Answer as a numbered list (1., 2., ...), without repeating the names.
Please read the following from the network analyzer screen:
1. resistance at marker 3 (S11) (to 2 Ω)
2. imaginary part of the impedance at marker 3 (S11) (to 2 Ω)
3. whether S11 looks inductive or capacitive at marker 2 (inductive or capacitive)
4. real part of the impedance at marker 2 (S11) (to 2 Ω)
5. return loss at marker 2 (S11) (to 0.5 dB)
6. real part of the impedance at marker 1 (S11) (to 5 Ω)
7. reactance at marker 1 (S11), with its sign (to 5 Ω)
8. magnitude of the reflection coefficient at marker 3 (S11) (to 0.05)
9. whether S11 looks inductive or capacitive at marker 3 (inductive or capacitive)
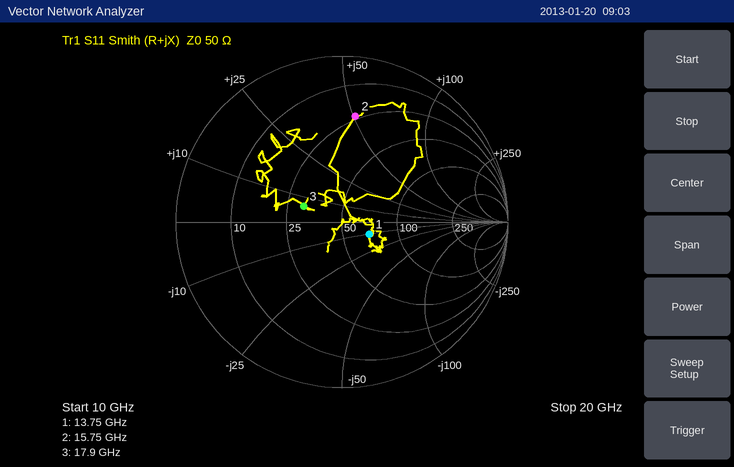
1. 30 Ω
2. +6 Ω
3. inductive
4. 24 Ω
5. 4.0 dB
6. 70 Ω
7. -10 Ω
8. 0.25
9. inductive
